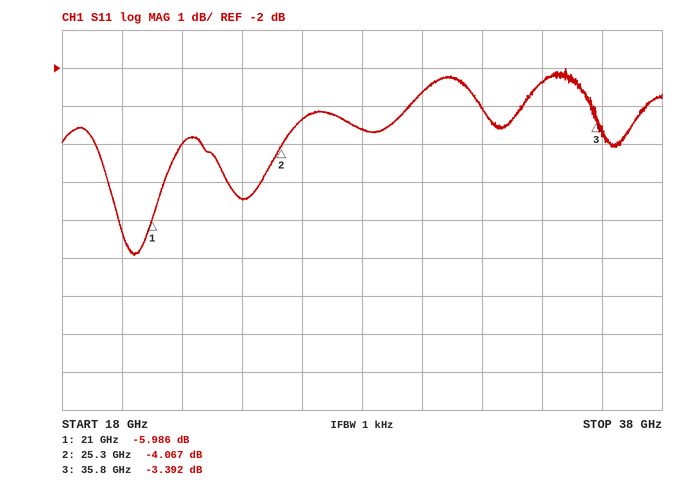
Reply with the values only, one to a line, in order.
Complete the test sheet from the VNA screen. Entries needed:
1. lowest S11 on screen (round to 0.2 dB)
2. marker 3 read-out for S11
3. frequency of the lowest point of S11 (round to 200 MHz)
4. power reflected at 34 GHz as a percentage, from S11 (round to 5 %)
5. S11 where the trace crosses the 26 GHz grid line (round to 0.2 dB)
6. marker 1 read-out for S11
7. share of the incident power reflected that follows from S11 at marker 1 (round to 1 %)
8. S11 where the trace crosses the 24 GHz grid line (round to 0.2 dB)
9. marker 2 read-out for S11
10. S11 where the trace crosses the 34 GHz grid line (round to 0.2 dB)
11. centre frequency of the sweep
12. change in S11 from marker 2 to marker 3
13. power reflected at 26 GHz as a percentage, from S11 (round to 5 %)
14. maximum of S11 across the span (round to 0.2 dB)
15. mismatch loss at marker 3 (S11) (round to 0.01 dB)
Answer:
-7.0 dB
-3.392 dB
20.4 GHz
60 %
-3.4 dB
-5.986 dB
25 %
-5.4 dB
-4.067 dB
-2.4 dB
28 GHz
0.675 dB
45 %
-2.0 dB
2.66 dB
